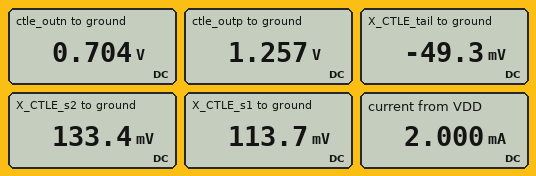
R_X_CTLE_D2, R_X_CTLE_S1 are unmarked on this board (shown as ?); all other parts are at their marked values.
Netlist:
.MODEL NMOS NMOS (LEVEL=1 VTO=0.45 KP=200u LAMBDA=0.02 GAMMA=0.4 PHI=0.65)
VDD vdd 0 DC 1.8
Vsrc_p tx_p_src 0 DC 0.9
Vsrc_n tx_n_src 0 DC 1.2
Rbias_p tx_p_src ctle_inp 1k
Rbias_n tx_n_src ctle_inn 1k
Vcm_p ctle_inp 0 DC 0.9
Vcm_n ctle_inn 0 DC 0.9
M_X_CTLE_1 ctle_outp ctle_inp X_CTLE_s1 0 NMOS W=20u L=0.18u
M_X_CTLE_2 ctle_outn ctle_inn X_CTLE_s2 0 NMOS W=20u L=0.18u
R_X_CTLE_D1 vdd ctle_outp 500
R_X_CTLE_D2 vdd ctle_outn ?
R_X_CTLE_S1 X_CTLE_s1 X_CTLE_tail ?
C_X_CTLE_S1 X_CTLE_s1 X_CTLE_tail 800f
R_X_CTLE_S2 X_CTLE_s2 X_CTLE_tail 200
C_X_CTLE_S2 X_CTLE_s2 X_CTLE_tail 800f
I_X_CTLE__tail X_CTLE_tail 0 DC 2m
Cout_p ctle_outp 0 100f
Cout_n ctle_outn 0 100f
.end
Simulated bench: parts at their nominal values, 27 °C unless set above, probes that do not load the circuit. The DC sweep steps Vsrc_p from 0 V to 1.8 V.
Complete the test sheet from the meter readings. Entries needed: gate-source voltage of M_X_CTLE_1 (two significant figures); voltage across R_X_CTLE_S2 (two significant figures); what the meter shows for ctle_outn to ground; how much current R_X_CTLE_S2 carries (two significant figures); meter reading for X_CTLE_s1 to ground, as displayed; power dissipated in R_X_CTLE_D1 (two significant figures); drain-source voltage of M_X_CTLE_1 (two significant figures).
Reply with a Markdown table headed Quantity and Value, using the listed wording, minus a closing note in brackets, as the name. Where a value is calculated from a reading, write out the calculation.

| Quantity | Value |
|---|---|
| gate-source voltage of M_X_CTLE_1 | 900 mV - 113.7 mV = 790 mV |
| voltage across R_X_CTLE_S2 | 133.4 mV - (-49.3 mV) = 180 mV |
| what the meter shows for ctle_outn to ground | 0.704 V |
| how much current R_X_CTLE_S2 carries | (133.4 mV - (-49.3 mV)) / 200 Ω = 910 µA |
| meter reading for X_CTLE_s1 to ground, as displayed | 113.7 mV |
| power dissipated in R_X_CTLE_D1 | (1.8 V - 1.257 V)^2 / 500 Ω = 590 µW |
| drain-source voltage of M_X_CTLE_1 | 1.257 V - 113.7 mV = 1.1 V |
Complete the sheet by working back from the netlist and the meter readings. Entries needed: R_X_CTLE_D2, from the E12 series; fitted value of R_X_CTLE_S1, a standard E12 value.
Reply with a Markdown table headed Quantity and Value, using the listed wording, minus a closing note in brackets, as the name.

| Quantity | Value |
|---|---|
| R_X_CTLE_D2, from the E12 series | 1.2 kΩ |
| fitted value of R_X_CTLE_S1, a standard E12 value | 150 Ω |
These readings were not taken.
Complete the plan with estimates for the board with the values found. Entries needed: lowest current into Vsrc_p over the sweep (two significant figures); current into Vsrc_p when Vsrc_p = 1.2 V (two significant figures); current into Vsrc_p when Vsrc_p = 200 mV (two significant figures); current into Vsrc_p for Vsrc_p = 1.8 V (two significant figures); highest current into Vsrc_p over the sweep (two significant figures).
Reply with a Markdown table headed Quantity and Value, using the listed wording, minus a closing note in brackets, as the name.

| Quantity | Value |
|---|---|
| lowest current into Vsrc_p over the sweep | -900 µA |
| current into Vsrc_p when Vsrc_p = 1.2 V | -300 µA |
| current into Vsrc_p when Vsrc_p = 200 mV | 700 µA |
| current into Vsrc_p for Vsrc_p = 1.8 V | -900 µA |
| highest current into Vsrc_p over the sweep | 900 µA |
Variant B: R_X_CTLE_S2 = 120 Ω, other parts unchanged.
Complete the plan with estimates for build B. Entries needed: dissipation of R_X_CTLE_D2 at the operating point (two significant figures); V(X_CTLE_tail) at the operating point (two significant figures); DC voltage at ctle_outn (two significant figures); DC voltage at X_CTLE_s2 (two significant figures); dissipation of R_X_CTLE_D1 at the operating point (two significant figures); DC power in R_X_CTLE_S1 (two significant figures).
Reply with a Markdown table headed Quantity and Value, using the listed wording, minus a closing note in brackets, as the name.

| Quantity | Value |
|---|---|
| dissipation of R_X_CTLE_D2 at the operating point | 1.3 mW |
| V(X_CTLE_tail) at the operating point | -11 mV |
| DC voltage at ctle_outn | 530 mV |
| DC voltage at X_CTLE_s2 | 120 mV |
| dissipation of R_X_CTLE_D1 at the operating point | 450 µW |
| DC power in R_X_CTLE_S1 | 130 µW |
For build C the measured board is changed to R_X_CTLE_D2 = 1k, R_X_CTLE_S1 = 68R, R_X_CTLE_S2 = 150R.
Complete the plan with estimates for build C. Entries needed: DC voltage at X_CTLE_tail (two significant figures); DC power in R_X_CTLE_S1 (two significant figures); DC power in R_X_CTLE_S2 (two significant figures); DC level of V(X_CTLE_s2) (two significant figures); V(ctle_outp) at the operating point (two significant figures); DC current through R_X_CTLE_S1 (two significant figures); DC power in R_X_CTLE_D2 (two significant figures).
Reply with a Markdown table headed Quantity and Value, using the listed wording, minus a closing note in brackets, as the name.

| Quantity | Value |
|---|---|
| DC voltage at X_CTLE_tail | 23 mV |
| DC power in R_X_CTLE_S1 | 95 µW |
| DC power in R_X_CTLE_S2 | 100 µW |
| DC level of V(X_CTLE_s2) | 150 mV |
| V(ctle_outp) at the operating point | 1.2 V |
| DC current through R_X_CTLE_S1 | 1.2 mA |
| DC power in R_X_CTLE_D2 | 670 µW |
